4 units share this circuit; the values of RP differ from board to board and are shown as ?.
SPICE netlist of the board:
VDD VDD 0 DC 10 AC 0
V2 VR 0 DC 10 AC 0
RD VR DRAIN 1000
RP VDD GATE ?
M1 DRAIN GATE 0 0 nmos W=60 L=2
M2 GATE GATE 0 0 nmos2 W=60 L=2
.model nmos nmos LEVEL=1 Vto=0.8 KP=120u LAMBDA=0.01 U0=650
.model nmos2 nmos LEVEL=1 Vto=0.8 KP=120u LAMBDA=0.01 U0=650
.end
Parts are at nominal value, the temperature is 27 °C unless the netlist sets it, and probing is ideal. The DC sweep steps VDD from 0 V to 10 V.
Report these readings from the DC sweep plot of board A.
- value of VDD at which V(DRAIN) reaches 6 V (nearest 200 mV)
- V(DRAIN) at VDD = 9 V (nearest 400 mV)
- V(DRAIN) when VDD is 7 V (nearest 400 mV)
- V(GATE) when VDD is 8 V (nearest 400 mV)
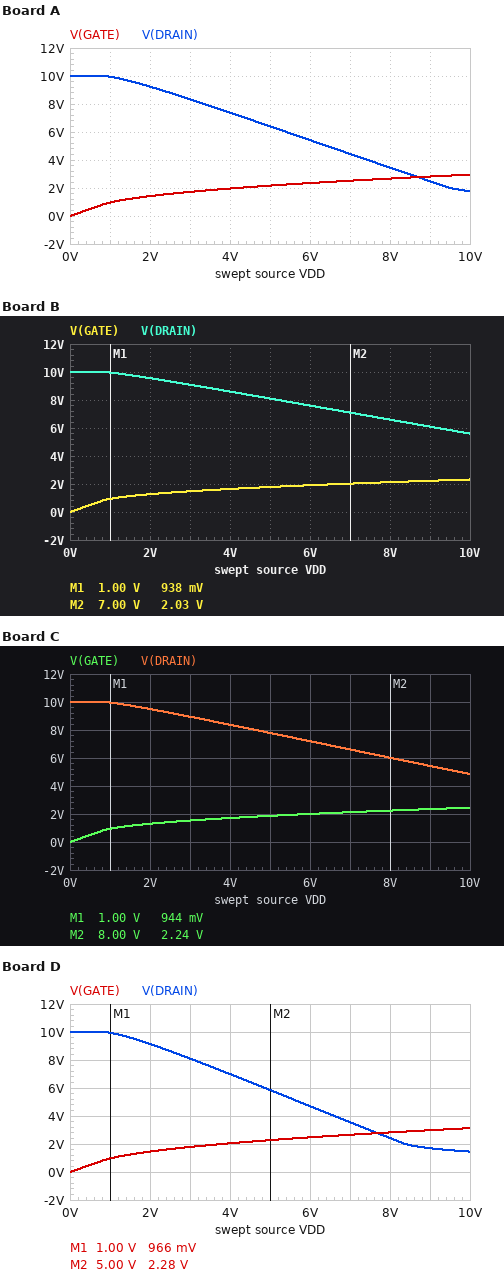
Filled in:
5.4 V
2.4 V
4.4 V
2.8 V
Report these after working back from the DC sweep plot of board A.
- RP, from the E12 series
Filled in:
820 Ω
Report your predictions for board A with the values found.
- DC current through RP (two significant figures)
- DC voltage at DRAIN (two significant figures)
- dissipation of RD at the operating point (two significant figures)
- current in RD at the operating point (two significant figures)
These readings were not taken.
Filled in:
8.6 mA
1.8 V
68 mW
8.2 mA
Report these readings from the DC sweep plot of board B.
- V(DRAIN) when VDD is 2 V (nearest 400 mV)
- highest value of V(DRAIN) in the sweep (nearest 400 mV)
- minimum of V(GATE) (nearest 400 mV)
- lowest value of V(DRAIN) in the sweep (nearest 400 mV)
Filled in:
9.6 V
10.0 V
0 V
5.6 V
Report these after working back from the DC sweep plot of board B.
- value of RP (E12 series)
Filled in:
1.8 kΩ
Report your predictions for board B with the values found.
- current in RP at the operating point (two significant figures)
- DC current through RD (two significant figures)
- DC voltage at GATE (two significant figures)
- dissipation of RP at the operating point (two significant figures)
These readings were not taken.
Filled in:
4.3 mA
4.4 mA
2.3 V
33 mW
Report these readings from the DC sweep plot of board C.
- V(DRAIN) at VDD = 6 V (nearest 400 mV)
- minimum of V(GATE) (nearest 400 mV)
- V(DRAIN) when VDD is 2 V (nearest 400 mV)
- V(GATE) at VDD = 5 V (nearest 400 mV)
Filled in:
7.2 V
0 V
9.6 V
2.0 V
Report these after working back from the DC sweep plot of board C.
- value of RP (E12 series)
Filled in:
1.5 kΩ
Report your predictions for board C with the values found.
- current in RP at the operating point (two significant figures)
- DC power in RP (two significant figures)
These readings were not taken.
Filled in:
5.0 mA
38 mW
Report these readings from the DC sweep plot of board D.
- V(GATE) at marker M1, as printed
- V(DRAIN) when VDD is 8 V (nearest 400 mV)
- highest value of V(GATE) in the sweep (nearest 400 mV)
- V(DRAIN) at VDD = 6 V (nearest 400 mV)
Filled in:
966 mV
2.4 V
3.2 V
4.8 V
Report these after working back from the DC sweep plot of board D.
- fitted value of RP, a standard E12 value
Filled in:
680 Ω
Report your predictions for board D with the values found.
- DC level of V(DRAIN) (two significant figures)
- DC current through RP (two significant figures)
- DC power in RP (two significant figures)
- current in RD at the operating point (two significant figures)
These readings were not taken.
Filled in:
1.5 V
10 mA
69 mW
8.5 mA
